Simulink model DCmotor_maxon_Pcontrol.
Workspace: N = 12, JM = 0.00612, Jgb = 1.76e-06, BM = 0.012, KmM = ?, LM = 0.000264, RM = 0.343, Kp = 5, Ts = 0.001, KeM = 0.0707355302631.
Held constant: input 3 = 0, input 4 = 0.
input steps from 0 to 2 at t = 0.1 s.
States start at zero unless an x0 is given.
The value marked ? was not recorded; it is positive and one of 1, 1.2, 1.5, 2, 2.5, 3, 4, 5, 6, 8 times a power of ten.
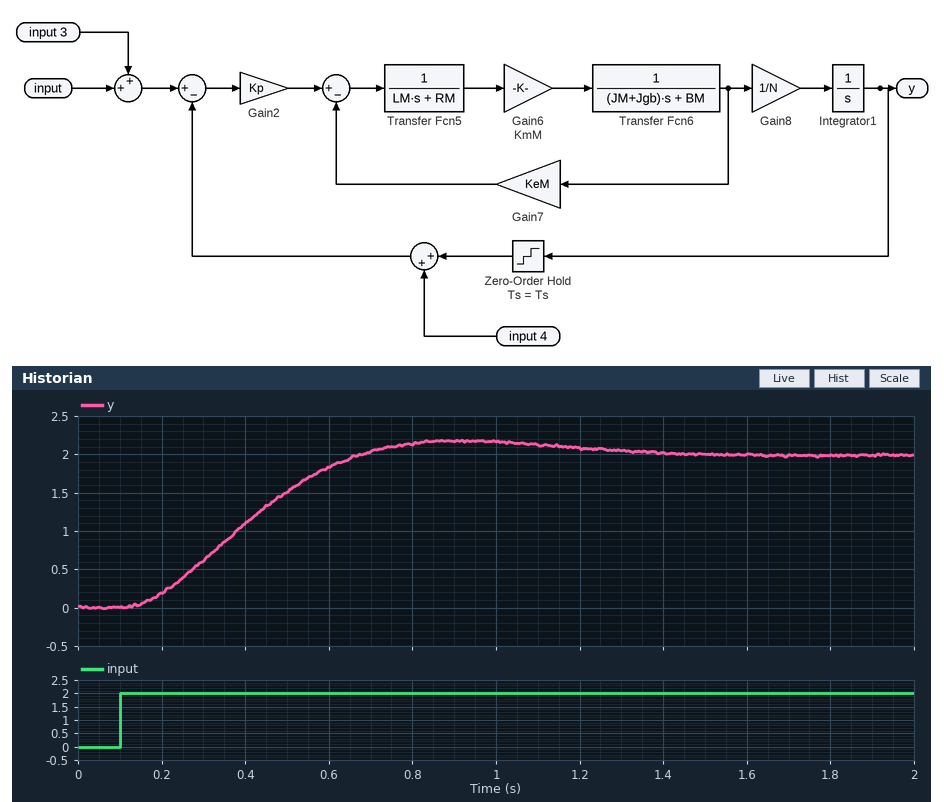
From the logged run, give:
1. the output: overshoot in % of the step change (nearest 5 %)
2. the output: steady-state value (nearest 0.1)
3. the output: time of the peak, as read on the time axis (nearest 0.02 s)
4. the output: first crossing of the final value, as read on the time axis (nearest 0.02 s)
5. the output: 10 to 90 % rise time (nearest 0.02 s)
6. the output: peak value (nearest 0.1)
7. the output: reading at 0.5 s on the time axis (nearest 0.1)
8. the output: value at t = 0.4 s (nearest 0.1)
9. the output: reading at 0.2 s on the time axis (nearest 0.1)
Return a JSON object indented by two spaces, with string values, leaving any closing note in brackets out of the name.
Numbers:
{
  "the output: overshoot in % of the step change": "10 %",
  "the output: steady-state value": "2.0",
  "the output: time of the peak, as read on the time axis": "0.92 s",
  "the output: first crossing of the final value, as read on the time axis": "0.68 s",
  "the output: 10 to 90 % rise time": "0.38 s",
  "the output: peak value": "2.2",
  "the output: reading at 0.5 s on the time axis": "1.5",
  "the output: value at t = 0.4 s": "1.1",
  "the output: reading at 0.2 s on the time axis": "0.2"
}
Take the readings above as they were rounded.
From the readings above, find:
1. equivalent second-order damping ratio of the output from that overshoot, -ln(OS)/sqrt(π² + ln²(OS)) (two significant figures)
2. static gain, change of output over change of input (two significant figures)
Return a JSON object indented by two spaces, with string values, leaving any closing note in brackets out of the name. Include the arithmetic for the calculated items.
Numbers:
{
  "equivalent second-order damping ratio of the output from that overshoot, -ln(OS)/sqrt(π² + ln²(OS))": "ln(0.1) = -2.303; 2.303 / sqrt(9.870 + 5.302) = 0.59",
  "static gain, change of output over change of input": "(2 - 0) / (2 - 0) = 1.0"
}
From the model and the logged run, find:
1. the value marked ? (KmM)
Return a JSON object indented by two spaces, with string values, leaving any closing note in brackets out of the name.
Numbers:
{
  "the value marked ?": "0.12"
}
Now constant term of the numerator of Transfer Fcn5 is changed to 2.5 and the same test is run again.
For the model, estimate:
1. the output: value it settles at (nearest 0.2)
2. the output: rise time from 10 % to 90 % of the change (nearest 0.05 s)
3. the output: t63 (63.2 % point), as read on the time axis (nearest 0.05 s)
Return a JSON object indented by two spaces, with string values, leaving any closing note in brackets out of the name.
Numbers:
{
  "the output: value it settles at": "2.0",
  "the output: rise time from 10 % to 90 % of the change": "0.30 s",
  "the output: t63 (63.2 % point), as read on the time axis": "0.35 s"
}
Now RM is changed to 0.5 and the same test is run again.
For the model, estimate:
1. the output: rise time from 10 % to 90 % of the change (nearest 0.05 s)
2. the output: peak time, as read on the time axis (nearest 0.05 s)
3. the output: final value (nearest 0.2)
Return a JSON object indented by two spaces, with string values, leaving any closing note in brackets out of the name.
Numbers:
{
  "the output: rise time from 10 % to 90 % of the change": "0.45 s",
  "the output: peak time, as read on the time axis": "1.05 s",
  "the output: final value": "2.0"
}
